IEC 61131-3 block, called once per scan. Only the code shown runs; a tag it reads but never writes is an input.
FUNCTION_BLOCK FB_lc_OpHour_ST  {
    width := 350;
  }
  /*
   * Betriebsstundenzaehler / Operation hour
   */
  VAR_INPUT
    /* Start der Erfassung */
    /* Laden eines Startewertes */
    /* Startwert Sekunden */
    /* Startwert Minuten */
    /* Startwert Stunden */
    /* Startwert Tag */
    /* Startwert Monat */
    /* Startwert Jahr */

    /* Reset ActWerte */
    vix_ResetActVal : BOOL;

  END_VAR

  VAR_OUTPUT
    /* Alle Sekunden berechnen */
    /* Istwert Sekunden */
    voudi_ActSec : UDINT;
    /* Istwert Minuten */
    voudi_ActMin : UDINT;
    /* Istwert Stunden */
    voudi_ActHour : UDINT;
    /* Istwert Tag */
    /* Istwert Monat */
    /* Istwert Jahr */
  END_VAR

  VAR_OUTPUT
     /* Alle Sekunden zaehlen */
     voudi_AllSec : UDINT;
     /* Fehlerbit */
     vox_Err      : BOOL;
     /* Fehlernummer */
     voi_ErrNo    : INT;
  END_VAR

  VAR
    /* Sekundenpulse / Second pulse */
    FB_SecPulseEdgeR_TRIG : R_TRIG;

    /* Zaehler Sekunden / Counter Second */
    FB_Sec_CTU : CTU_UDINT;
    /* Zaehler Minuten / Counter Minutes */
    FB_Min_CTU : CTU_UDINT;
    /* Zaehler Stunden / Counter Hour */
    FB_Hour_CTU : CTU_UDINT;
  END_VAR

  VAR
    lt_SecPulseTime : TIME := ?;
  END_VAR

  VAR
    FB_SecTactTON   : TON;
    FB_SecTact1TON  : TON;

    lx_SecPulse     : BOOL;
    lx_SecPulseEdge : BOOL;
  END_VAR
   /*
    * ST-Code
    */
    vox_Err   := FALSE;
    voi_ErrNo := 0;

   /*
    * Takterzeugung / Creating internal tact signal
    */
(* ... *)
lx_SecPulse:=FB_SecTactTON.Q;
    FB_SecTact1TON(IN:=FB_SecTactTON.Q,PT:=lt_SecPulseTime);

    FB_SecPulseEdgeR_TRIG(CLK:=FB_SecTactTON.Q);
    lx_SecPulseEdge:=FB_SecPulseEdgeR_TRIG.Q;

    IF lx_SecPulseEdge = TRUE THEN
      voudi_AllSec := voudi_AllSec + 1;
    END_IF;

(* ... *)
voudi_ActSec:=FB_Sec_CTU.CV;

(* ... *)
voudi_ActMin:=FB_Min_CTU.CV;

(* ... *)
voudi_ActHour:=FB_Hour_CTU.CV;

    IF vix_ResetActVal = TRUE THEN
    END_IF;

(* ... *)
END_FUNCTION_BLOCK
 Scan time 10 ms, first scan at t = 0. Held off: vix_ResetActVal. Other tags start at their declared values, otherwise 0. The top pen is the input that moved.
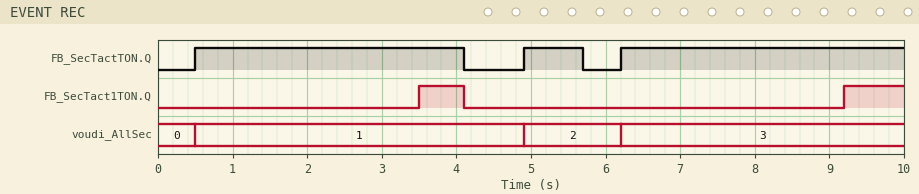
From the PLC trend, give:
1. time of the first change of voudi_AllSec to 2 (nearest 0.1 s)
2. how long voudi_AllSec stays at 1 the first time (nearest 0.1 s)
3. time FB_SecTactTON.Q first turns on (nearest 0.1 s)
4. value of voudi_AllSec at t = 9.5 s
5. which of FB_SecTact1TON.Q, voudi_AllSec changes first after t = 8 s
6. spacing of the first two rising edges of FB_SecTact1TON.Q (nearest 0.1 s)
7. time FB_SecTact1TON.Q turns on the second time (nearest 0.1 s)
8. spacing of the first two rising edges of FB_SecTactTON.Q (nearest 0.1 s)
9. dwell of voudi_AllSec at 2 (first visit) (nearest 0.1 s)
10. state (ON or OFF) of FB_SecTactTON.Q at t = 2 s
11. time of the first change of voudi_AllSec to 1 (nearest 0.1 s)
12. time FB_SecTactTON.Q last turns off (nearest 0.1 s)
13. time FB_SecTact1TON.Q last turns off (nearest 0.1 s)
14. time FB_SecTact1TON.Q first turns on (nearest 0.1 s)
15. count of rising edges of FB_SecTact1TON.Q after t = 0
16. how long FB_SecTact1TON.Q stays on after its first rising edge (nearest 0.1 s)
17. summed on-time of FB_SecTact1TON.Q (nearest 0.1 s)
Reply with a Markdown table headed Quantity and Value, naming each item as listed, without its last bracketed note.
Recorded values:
| Quantity | Value |
|---|---|
| time of the first change of voudi_AllSec to 2 | 4.9 s |
| how long voudi_AllSec stays at 1 the first time | 4.4 s |
| time FB_SecTactTON.Q first turns on | 0.5 s |
| value of voudi_AllSec at t = 9.5 s | 3 |
| which of FB_SecTact1TON.Q, voudi_AllSec changes first after t = 8 s | FB_SecTact1TON.Q |
| spacing of the first two rising edges of FB_SecTact1TON.Q | 5.7 s |
| time FB_SecTact1TON.Q turns on the second time | 9.2 s |
| spacing of the first two rising edges of FB_SecTactTON.Q | 4.4 s |
| dwell of voudi_AllSec at 2 (first visit) | 1.3 s |
| state (ON or OFF) of FB_SecTactTON.Q at t = 2 s | ON |
| time of the first change of voudi_AllSec to 1 | 0.5 s |
| time FB_SecTactTON.Q last turns off | 5.7 s |
| time FB_SecTact1TON.Q last turns off | 4.1 s |
| time FB_SecTact1TON.Q first turns on | 3.5 s |
| count of rising edges of FB_SecTact1TON.Q after t = 0 | 2 |
| how long FB_SecTact1TON.Q stays on after its first rising edge | 0.6 s |
| summed on-time of FB_SecTact1TON.Q | 1.4 s |
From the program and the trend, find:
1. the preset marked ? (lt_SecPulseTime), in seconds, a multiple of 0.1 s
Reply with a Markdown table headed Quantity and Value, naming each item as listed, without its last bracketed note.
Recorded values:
| Quantity | Value |
|---|---|
| the preset marked ? (lt_SecPulseTime), in seconds, a multiple of 0.1 s | 3.0 s |
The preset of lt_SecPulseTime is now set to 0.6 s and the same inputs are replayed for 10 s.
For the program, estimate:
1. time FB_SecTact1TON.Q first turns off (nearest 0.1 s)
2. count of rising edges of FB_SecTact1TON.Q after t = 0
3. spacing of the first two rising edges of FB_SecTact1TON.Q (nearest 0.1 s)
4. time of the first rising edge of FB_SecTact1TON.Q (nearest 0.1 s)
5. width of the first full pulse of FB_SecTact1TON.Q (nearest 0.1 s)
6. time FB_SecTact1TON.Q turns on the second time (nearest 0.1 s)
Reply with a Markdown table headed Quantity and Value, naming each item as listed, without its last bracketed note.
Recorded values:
| Quantity | Value |
|---|---|
| time FB_SecTact1TON.Q first turns off | 4.1 s |
| count of rising edges of FB_SecTact1TON.Q after t = 0 | 3 |
| spacing of the first two rising edges of FB_SecTact1TON.Q | 4.4 s |
| time of the first rising edge of FB_SecTact1TON.Q | 1.1 s |
| width of the first full pulse of FB_SecTact1TON.Q | 3.0 s |
| time FB_SecTact1TON.Q turns on the second time | 5.5 s |
